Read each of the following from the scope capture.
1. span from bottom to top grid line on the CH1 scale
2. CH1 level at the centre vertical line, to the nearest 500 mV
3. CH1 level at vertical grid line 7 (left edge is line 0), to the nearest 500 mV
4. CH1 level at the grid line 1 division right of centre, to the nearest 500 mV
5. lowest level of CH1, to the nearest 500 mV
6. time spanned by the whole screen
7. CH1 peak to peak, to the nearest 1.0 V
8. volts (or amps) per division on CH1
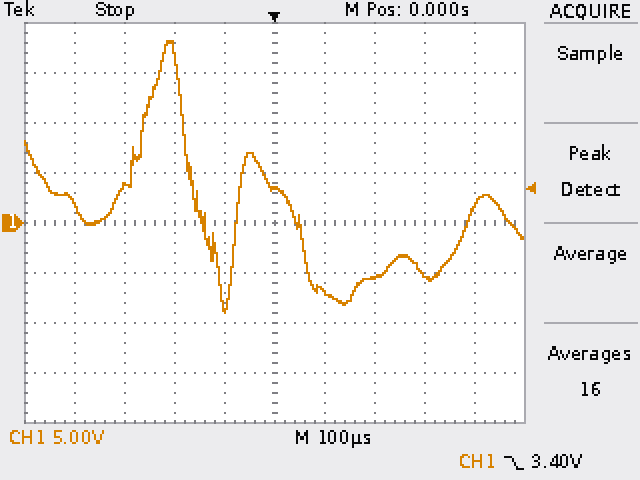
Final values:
40 V
3.5 V
-5.5 V
-7.0 V
-9.0 V
1 ms
27.0 V
5 V
